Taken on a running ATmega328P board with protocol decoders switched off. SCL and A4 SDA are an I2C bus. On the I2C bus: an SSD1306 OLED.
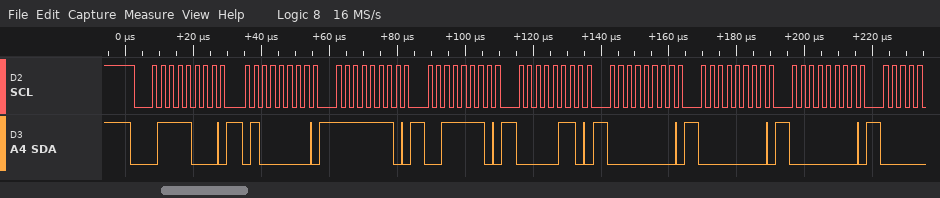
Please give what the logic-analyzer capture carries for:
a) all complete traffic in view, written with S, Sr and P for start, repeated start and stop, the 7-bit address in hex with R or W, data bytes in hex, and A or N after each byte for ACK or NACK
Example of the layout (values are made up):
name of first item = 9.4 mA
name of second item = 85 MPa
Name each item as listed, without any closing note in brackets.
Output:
all complete traffic in view, written with S, Sr and P for start, repeated start and stop, the 7-bit address in hex with R or W, data bytes in hex, and A or N after each byte for ACK or NACK = S 3CW A 40 A FE A 3E A 06 A 00 A 00 A 00 A
